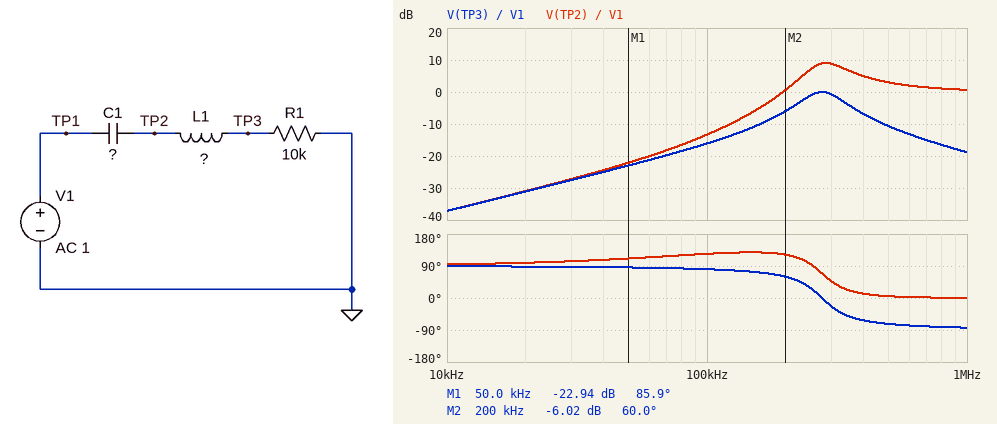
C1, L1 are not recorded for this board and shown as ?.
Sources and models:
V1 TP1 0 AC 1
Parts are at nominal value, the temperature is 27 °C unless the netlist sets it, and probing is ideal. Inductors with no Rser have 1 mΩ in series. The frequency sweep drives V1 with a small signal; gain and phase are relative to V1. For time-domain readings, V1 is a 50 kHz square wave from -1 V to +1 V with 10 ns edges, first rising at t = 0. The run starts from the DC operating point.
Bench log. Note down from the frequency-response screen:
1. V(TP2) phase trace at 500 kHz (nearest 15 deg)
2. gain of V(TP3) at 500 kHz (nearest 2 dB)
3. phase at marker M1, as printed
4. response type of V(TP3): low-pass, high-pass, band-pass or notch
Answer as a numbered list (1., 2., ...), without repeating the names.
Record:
1. 0 deg
2. -10 dB
3. 85.9 deg
4. band-pass
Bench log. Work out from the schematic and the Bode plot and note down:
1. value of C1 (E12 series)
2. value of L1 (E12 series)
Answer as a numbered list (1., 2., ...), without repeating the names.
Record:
1. 22 pF
2. 15 mH
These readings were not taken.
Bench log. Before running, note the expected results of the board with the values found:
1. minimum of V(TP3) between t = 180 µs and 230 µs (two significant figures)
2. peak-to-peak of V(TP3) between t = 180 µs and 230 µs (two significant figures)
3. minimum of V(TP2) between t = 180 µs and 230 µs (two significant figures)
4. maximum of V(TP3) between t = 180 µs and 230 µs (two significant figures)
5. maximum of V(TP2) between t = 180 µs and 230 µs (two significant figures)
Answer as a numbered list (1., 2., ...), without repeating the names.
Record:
1. -590 mV
2. 1.2 V
3. -2.0 V
4. 590 mV
5. 2.0 V
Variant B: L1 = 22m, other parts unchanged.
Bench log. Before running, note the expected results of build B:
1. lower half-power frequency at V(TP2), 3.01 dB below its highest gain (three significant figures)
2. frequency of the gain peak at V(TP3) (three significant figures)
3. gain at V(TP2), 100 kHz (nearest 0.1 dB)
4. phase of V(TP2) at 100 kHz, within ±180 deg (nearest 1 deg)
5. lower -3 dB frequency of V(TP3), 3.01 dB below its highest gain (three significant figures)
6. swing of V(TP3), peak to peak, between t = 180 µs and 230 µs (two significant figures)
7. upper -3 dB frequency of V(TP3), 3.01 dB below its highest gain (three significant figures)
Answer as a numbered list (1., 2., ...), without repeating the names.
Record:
1. 203 kHz
2. 229 kHz
3. -10.8 dB
4. 134 deg
5. 195 kHz
6. 990 mV
7. 268 kHz
